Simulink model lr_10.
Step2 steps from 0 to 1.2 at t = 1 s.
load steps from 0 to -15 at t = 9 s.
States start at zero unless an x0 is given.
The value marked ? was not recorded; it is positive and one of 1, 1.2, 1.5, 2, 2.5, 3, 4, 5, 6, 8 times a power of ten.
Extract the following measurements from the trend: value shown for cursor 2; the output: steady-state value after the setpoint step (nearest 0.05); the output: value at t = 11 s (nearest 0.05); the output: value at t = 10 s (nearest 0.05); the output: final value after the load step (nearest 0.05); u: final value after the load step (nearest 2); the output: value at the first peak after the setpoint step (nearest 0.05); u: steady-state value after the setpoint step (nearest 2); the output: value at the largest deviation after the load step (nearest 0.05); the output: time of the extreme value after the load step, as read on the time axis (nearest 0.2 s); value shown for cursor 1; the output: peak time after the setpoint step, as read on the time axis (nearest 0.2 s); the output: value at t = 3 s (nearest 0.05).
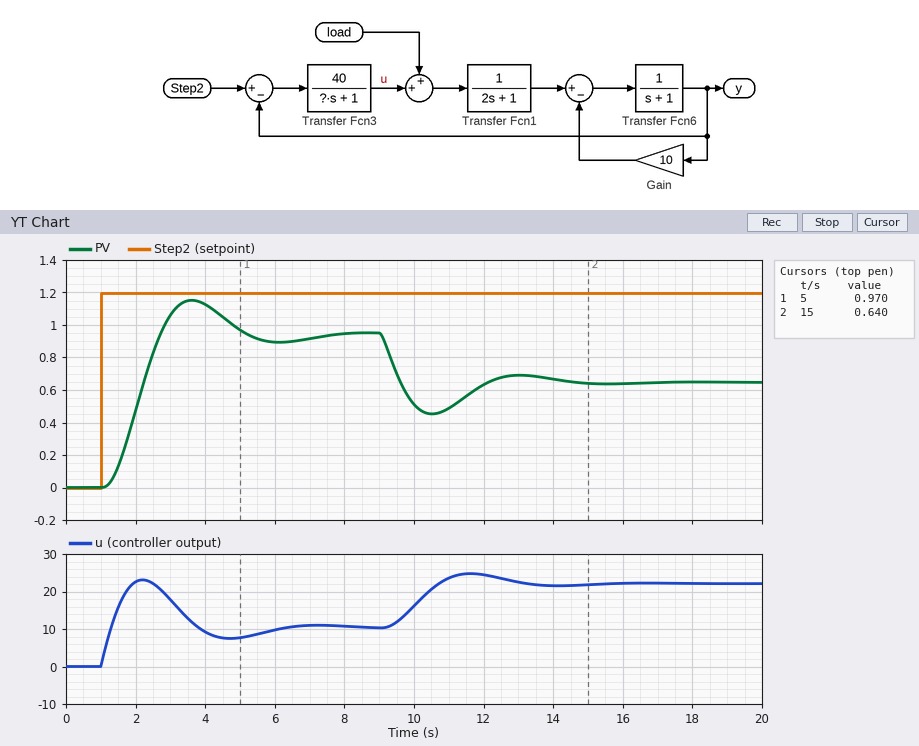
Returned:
0.640
0.95
0.50
0.50
0.65
22
1.15
10
0.45
10.6 s
0.970
3.6 s
1.05
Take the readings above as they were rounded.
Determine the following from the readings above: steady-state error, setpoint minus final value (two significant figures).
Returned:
0.25
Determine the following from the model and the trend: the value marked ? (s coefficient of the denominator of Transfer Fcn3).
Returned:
1.2
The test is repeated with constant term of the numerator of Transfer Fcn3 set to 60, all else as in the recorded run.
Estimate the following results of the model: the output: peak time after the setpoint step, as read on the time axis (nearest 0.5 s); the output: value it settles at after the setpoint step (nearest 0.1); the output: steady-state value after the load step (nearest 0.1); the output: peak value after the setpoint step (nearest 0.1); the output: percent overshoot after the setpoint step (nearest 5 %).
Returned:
3.0 s
1.0
0.8
1.3
30 %
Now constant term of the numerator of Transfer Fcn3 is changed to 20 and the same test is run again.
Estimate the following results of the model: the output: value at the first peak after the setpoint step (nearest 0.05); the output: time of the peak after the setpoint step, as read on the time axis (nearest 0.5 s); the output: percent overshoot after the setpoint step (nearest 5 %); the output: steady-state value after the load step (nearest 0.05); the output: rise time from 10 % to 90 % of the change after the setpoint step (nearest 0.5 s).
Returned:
0.85
4.5 s
10 %
0.30
1.5 s
